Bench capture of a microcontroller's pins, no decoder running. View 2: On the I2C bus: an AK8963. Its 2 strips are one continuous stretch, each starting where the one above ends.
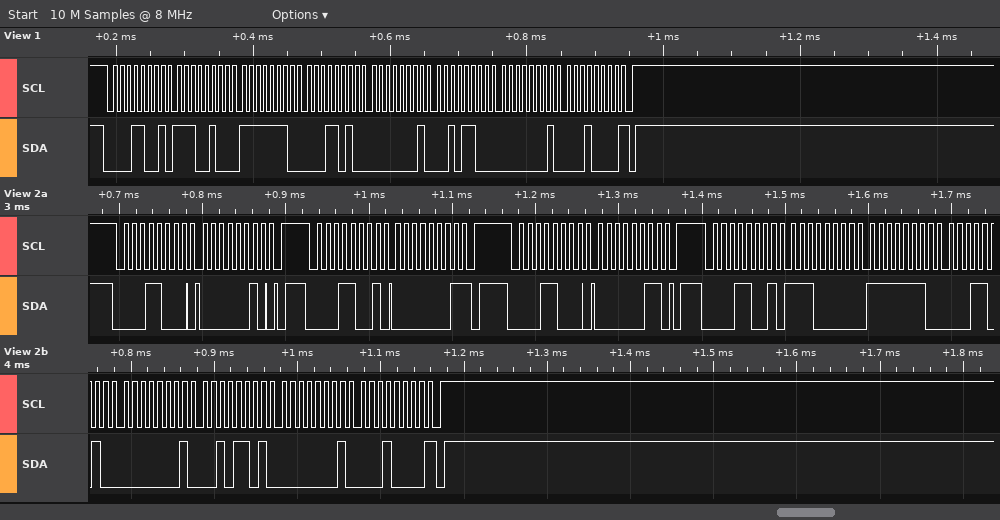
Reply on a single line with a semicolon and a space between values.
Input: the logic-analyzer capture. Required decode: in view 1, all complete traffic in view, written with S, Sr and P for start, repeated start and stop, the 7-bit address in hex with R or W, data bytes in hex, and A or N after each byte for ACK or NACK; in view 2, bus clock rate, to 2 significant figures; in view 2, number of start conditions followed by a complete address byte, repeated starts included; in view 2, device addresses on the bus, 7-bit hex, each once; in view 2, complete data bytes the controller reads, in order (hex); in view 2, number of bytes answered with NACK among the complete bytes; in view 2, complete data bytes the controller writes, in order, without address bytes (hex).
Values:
S 0CR A E4 A FE A 1A A 01 A 2C A 01 A 10 N P; 100 kHz; 4; 0x0C; 01 E0 FE 1A 01 2D 01 10; 2; 02 03
